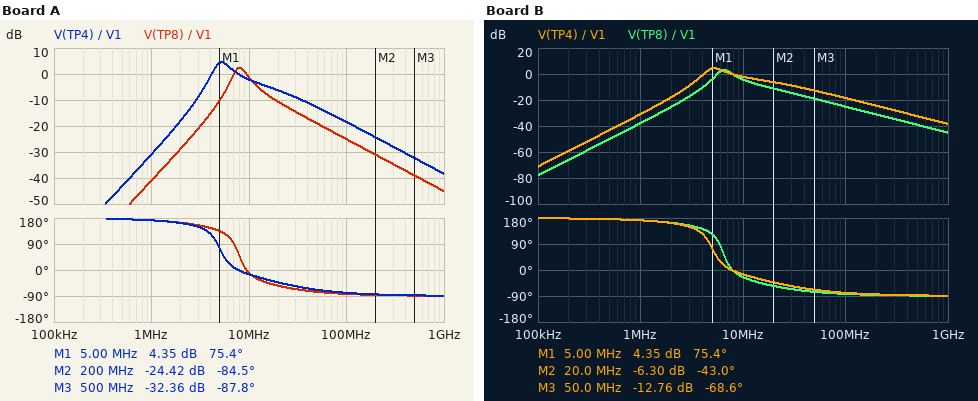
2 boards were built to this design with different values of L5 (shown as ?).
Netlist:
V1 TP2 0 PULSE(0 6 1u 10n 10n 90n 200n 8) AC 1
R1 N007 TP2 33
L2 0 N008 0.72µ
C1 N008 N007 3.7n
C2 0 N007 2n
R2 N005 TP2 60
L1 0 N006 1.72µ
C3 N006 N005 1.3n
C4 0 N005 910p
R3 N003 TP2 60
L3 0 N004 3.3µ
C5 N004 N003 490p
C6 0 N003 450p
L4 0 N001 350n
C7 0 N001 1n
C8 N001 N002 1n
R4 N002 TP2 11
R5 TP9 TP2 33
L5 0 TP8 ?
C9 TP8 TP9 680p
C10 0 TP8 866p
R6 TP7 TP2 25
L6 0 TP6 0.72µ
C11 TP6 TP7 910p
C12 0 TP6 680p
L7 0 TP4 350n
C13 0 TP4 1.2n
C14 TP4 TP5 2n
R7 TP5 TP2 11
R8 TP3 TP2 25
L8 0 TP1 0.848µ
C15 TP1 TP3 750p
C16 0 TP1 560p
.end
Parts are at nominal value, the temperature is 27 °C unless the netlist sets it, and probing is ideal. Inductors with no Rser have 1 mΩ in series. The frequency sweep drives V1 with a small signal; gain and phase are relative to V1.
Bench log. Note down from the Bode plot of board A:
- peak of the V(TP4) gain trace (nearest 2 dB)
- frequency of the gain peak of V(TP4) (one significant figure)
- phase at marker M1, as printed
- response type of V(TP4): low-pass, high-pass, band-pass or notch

4 dB
5 MHz
75.4 deg
band-pass
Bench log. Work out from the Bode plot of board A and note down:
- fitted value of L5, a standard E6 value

330 nH
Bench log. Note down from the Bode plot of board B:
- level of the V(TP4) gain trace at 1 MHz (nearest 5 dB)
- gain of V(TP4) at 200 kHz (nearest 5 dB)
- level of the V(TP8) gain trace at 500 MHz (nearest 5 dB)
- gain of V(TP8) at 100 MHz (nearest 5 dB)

-30 dB
-60 dB
-40 dB
-25 dB
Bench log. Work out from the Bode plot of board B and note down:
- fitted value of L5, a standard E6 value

470 nH
